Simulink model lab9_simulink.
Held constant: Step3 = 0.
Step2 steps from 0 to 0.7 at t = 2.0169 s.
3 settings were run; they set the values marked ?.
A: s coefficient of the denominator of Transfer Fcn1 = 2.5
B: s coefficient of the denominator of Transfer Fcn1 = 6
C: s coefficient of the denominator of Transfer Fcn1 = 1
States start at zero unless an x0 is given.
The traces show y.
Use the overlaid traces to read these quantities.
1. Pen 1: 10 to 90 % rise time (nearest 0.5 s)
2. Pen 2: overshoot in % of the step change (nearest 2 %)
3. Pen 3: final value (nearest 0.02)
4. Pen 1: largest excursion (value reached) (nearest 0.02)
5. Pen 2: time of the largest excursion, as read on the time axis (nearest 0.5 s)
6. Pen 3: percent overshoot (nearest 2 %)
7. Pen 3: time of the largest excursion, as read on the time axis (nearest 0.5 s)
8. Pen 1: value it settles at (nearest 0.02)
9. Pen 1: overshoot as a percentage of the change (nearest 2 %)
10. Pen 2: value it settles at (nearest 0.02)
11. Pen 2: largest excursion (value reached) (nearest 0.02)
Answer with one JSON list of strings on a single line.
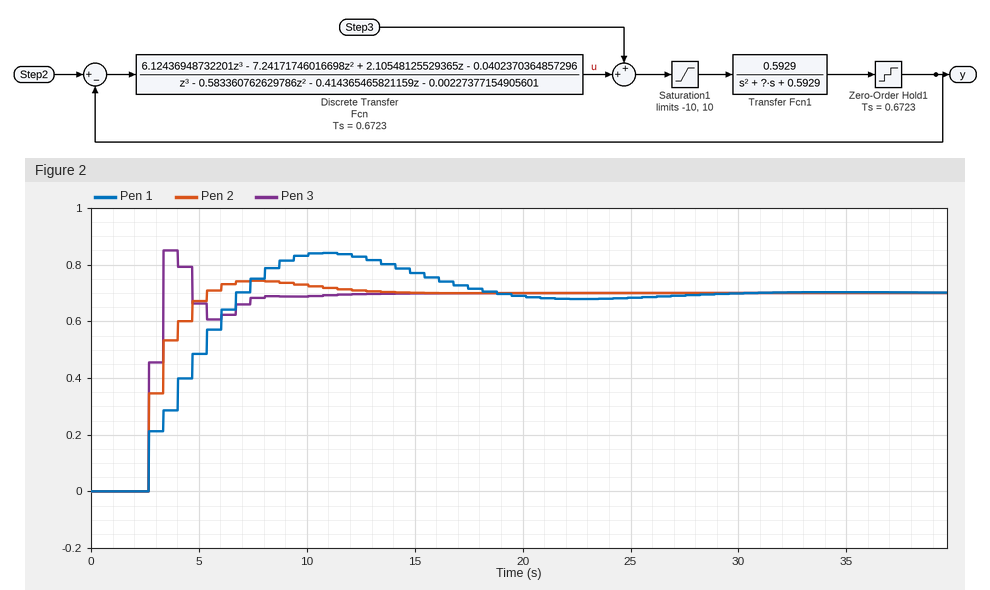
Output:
["3.5 s", "6 %", "0.70", "0.84", "7.5 s", "22 %", "3.5 s", "0.70", "20 %", "0.70", "0.74"]
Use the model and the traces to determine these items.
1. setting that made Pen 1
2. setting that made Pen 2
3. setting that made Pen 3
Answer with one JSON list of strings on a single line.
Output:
["B", "A", "C"]
